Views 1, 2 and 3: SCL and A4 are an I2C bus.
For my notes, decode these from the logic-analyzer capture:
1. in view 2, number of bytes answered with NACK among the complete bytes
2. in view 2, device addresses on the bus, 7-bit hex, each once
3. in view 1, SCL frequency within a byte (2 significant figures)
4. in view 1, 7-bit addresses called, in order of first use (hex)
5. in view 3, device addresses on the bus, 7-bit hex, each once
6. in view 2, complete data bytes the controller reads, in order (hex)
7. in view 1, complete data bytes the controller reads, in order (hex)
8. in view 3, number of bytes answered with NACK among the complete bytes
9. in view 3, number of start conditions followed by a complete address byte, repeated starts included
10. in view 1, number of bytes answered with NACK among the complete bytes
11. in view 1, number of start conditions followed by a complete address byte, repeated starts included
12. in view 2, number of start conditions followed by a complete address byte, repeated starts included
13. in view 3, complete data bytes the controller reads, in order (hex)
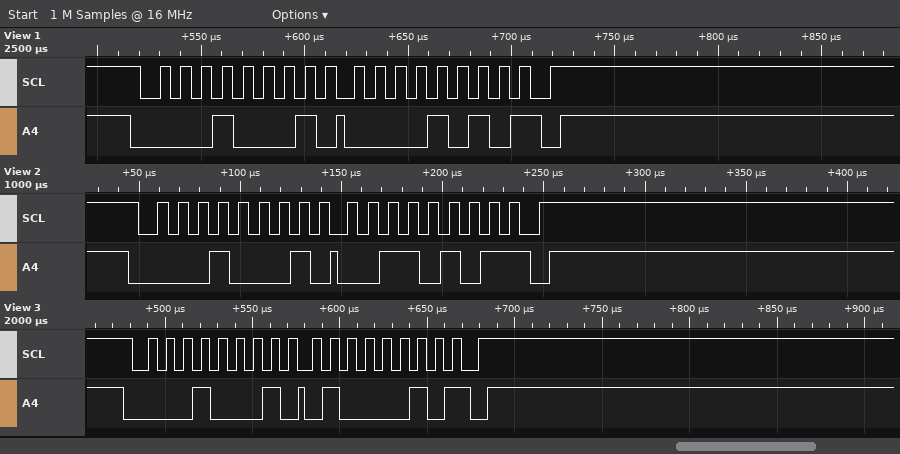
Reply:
1
0x08
100 kHz
0x08
0x08
35
0A
1
1
1
1
1
42
